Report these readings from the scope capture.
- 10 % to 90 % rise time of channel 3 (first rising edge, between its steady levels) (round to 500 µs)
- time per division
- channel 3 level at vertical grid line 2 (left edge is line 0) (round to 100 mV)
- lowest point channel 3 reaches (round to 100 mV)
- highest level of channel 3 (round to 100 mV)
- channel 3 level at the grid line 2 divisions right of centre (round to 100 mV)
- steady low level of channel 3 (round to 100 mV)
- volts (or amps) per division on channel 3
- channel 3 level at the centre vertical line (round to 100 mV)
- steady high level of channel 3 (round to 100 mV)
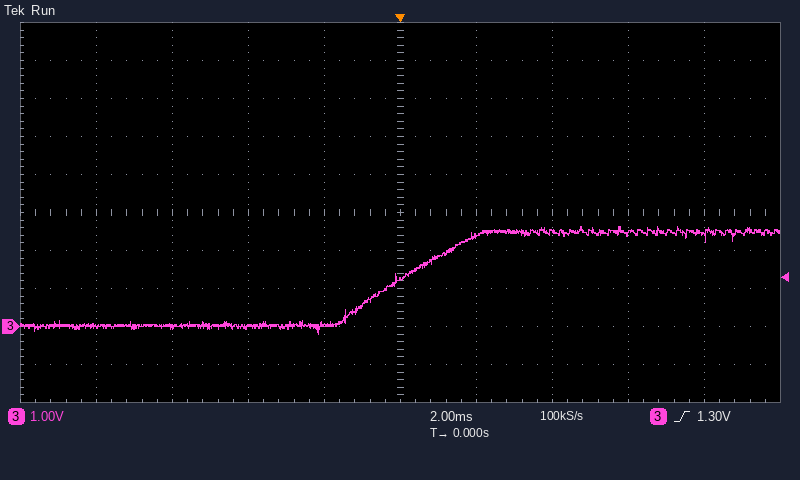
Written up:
3.0 ms
2 ms
0.0 V
-200 mV
2.6 V
2.5 V
0.0 V
1 V
1.2 V
2.5 V
